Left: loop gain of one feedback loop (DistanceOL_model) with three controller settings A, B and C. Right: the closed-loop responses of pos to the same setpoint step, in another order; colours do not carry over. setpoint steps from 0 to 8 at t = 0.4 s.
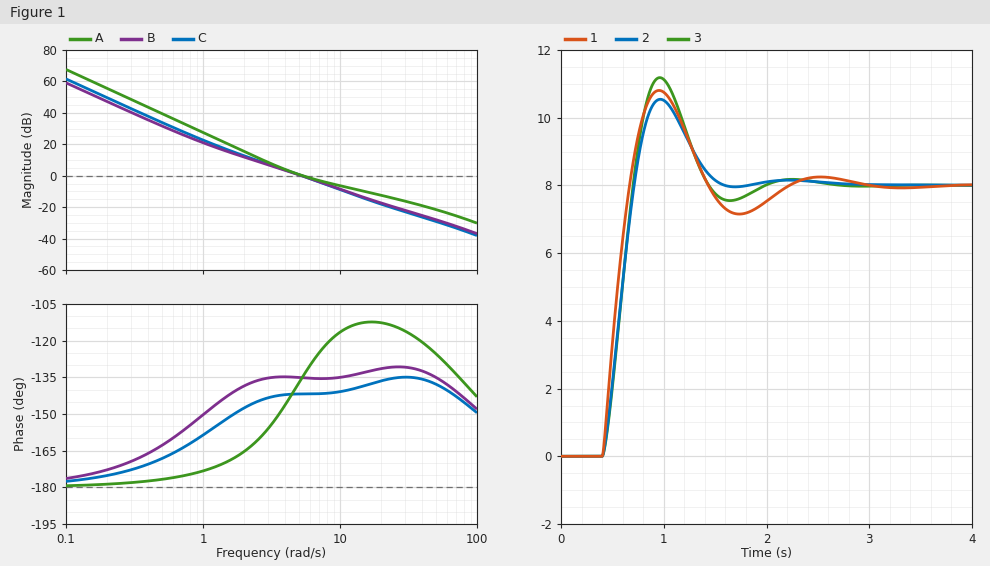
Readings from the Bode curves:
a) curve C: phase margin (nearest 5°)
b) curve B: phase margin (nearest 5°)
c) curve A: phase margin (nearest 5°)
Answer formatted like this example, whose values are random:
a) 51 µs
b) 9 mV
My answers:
a) 40°
b) 45°
c) 45°
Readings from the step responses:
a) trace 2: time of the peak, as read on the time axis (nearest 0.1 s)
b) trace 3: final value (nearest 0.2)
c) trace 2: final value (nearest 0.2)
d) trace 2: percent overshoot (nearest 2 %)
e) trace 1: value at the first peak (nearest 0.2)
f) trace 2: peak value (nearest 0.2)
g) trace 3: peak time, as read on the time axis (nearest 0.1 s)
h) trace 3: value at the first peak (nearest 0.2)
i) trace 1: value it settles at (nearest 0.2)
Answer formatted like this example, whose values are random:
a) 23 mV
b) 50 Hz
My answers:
a) 1.0 s
b) 8.0
c) 8.0
d) 32 %
e) 10.8
f) 10.6
g) 1.0 s
h) 11.2
i) 8.0
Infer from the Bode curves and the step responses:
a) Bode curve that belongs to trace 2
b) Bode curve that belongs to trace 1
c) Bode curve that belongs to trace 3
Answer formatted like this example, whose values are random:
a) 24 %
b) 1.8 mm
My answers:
a) B
b) A
c) C
